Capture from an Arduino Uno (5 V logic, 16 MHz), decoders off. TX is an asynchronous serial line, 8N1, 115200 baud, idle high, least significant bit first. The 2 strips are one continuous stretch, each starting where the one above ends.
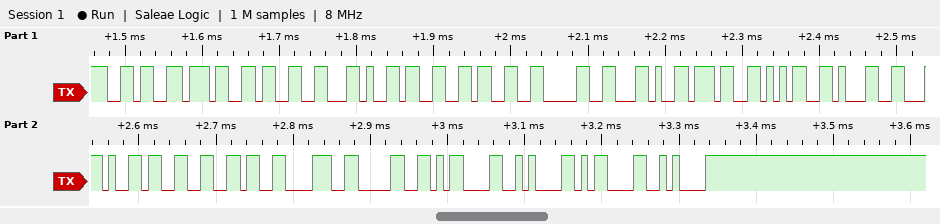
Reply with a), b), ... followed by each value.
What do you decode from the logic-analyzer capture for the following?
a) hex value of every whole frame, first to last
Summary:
a) 0x36 0x37 0x33 0x2C 0x33 0x33 0x30 0x2C 0x37 0x35 0x31 0x2C 0x33 0x36 0x38 0x30 0x0D 0x0A 0x0D 0x0A
